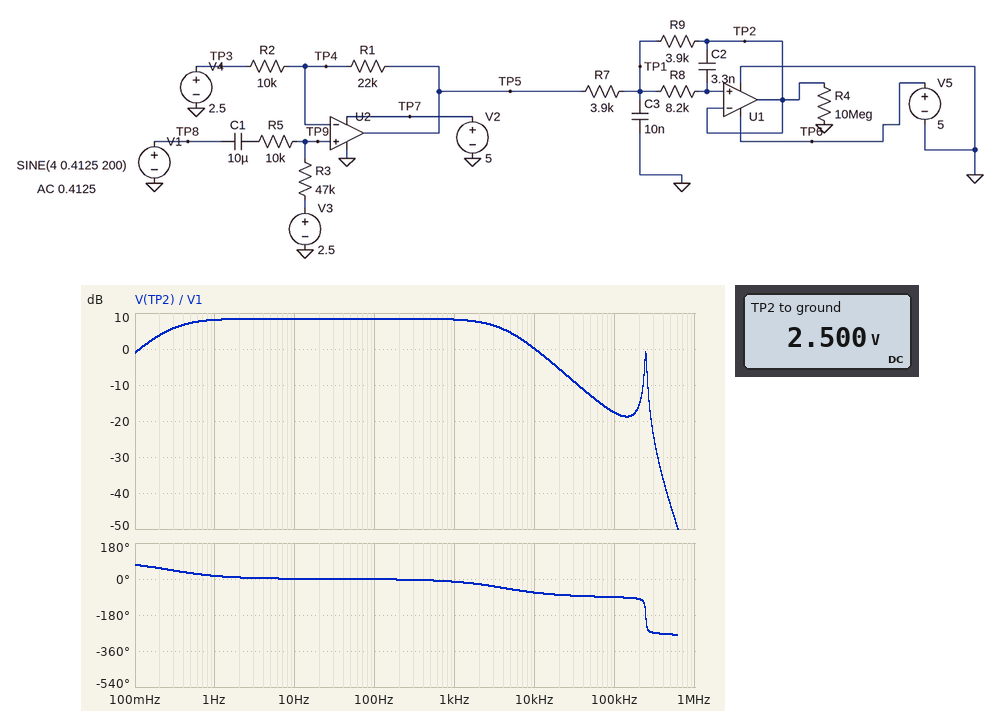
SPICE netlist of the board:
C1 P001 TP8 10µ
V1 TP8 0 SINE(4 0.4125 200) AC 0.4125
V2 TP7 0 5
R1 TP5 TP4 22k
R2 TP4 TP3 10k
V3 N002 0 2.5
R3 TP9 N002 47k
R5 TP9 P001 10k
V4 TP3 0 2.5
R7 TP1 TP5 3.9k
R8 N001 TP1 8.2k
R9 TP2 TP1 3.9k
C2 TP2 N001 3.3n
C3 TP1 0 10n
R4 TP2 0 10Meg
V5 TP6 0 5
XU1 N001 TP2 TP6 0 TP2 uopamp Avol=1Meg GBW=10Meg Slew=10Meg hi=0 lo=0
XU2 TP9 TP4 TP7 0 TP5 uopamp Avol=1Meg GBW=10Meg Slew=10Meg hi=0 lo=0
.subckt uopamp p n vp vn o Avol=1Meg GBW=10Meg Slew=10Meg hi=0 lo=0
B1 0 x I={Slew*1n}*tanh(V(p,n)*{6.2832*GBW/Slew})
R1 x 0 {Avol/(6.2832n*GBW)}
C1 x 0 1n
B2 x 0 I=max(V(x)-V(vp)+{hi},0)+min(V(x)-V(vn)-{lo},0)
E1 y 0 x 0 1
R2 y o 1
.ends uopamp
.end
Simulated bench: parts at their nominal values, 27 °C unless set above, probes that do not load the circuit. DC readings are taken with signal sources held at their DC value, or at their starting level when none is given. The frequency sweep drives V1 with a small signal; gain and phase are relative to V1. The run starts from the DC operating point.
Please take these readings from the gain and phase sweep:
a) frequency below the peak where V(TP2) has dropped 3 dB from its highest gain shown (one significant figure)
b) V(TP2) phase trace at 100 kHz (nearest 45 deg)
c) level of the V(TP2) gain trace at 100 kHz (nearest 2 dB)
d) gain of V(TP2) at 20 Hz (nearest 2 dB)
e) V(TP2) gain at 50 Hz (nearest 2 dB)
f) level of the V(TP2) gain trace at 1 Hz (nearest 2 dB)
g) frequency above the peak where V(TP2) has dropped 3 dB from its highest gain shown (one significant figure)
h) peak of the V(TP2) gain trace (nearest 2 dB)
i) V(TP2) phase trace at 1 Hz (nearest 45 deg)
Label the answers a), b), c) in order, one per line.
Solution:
a) 300 mHz
b) -90 deg
c) -18 dB
d) 8 dB
e) 8 dB
f) 8 dB
g) 4 kHz
h) 8 dB
i) 0 deg
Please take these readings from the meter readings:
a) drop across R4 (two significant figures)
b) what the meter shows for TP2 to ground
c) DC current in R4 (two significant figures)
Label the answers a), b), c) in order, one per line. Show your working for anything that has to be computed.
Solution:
a) 2.5 V = 2.5 V
b) 2.500 V
c) (2.5 V) / 10 MΩ = 250 nA
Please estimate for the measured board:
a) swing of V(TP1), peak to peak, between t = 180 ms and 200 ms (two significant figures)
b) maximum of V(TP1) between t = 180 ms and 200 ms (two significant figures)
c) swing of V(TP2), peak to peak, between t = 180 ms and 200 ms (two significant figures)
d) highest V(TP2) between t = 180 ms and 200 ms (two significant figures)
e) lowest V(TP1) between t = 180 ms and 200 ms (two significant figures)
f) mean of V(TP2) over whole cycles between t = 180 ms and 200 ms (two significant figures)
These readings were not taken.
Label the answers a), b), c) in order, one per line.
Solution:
a) 2.2 V
b) 3.6 V
c) 2.2 V
d) 3.6 V
e) 1.4 V
f) 2.5 V
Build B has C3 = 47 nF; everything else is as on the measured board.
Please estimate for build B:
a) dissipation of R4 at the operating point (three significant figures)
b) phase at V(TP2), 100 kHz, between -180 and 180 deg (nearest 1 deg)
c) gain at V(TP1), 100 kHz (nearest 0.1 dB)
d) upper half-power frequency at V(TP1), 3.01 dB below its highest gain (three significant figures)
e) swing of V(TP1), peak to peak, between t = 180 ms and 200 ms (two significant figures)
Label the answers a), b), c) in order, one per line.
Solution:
a) 625 nW
b) -92 deg
c) -32.8 dB
d) 869 Hz
e) 2.1 V
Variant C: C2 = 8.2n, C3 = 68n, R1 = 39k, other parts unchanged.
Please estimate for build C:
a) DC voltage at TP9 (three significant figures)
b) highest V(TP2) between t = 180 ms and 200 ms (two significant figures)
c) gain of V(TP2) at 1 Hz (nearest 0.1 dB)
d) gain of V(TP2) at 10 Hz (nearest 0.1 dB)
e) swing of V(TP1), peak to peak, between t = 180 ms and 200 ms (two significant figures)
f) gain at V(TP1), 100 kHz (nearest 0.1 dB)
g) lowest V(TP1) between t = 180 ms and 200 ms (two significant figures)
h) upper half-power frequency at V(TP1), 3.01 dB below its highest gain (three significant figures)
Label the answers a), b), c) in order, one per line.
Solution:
a) 2.50 V
b) 4.1 V
c) 11.8 dB
d) 12.1 dB
e) 3.2 V
f) -32.3 dB
g) 920 mV
h) 601 Hz
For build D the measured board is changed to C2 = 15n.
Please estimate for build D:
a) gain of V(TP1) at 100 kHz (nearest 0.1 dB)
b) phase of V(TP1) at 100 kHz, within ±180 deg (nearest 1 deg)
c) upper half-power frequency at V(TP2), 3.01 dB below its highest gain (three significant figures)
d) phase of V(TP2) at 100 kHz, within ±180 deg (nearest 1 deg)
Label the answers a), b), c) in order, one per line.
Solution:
a) -19.6 dB
b) -101 deg
c) 4.10 kHz
d) -104 deg
